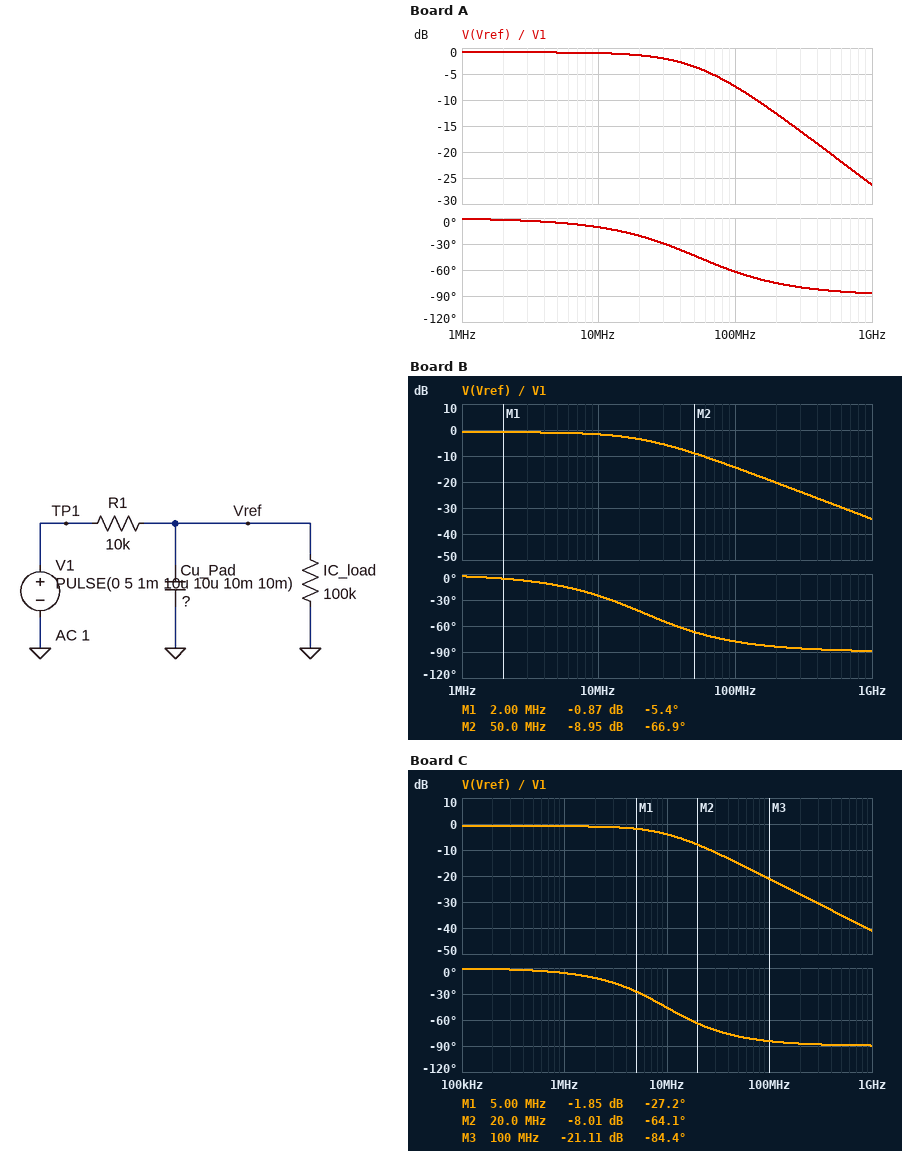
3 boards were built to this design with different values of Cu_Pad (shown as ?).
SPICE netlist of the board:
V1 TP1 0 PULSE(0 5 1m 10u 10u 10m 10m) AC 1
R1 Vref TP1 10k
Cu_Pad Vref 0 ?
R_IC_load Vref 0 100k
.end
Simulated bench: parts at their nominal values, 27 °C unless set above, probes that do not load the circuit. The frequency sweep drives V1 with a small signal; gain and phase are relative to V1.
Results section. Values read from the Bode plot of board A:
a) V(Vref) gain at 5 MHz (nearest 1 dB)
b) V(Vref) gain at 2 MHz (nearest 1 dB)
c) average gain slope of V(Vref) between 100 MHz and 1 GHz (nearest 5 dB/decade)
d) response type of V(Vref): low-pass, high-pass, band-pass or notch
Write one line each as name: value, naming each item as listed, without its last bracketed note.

V(Vref) gain at 5 MHz: -1 dB
V(Vref) gain at 2 MHz: -1 dB
average gain slope of V(Vref) between 100 MHz and 1 GHz: -20 dB/decade
response type of V(Vref): low-pass, high-pass, band-pass or notch: low-pass
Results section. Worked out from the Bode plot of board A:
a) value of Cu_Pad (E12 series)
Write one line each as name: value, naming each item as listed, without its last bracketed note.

value of Cu_Pad: 330 fF
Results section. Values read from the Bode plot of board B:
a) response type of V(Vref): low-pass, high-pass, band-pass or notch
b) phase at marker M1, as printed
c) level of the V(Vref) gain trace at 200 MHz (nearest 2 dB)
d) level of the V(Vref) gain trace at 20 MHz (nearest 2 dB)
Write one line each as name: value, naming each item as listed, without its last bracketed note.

response type of V(Vref): low-pass, high-pass, band-pass or notch: low-pass
phase at marker M1, as printed: -5.4 deg
level of the V(Vref) gain trace at 200 MHz: -20 dB
level of the V(Vref) gain trace at 20 MHz: -4 dB
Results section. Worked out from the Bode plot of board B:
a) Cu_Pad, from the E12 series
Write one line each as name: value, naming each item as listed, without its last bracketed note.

Cu_Pad, from the E12 series: 820 fF
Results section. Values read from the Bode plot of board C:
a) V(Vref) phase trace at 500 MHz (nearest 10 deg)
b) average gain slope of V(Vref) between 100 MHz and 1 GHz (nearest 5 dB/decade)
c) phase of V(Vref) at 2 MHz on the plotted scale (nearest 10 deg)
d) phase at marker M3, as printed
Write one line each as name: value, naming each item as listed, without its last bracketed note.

V(Vref) phase trace at 500 MHz: -90 deg
average gain slope of V(Vref) between 100 MHz and 1 GHz: -20 dB/decade
phase of V(Vref) at 2 MHz on the plotted scale: -10 deg
phase at marker M3, as printed: -84.4 deg
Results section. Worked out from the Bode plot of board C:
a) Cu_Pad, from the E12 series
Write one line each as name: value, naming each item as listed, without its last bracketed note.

Cu_Pad, from the E12 series: 1.8 pF
